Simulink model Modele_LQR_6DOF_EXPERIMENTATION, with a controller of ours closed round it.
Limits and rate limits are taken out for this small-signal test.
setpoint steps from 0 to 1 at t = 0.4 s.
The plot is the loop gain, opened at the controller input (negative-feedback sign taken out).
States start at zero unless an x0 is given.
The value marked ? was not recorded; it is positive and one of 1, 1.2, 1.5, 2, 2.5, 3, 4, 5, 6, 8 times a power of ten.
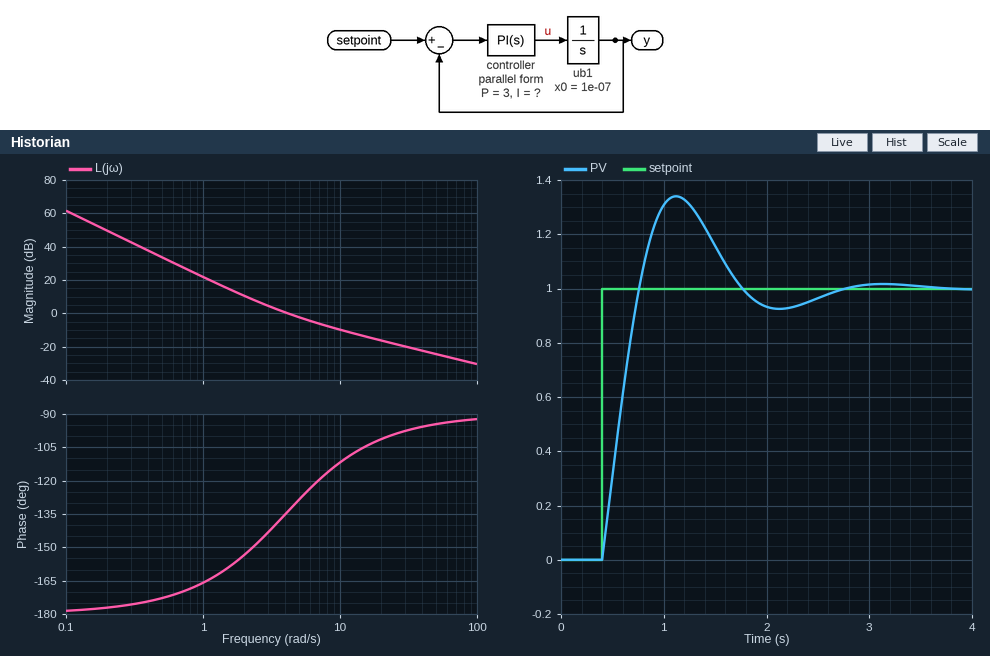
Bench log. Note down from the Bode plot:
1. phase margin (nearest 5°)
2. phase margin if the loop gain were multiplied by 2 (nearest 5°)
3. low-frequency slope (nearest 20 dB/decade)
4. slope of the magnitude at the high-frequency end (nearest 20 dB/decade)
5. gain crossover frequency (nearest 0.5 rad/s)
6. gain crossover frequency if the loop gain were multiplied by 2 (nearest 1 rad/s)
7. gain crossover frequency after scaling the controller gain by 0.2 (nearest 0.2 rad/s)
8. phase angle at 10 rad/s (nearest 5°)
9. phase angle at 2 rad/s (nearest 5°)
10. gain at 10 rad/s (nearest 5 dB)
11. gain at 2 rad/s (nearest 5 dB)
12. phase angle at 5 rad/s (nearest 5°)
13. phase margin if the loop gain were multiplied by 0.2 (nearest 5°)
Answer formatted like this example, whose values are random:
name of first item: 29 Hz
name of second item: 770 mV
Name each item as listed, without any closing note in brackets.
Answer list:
phase margin: 45°
phase margin if the loop gain were multiplied by 2: 60°
low-frequency slope: -40 dB/decade
slope of the magnitude at the high-frequency end: -20 dB/decade
gain crossover frequency: 4.0 rad/s
gain crossover frequency if the loop gain were multiplied by 2: 7 rad/s
gain crossover frequency after scaling the controller gain by 0.2: 1.6 rad/s
phase angle at 10 rad/s: -110°
phase angle at 2 rad/s: -155°
gain at 10 rad/s: -10 dB
gain at 2 rad/s: 10 dB
phase angle at 5 rad/s: -130°
phase margin if the loop gain were multiplied by 0.2: 20°
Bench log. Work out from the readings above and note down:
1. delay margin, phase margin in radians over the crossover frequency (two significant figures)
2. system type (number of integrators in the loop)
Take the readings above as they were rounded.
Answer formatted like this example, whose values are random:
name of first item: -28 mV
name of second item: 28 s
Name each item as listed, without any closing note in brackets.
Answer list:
delay margin, phase margin in radians over the crossover frequency: 0.20 s
system type: 2
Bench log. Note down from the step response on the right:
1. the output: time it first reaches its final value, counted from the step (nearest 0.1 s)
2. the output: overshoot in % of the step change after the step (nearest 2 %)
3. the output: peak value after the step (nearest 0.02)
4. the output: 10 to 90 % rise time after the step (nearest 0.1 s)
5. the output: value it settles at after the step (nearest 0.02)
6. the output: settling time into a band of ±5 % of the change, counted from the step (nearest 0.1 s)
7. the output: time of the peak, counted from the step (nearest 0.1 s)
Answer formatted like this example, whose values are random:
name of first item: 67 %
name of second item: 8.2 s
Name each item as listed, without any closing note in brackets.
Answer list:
the output: time it first reaches its final value, counted from the step: 0.4 s
the output: overshoot in % of the step change after the step: 34 %
the output: peak value after the step: 1.34
the output: 10 to 90 % rise time after the step: 0.3 s
the output: value it settles at after the step: 1.00
the output: settling time into a band of ±5 % of the change, counted from the step: 2.0 s
the output: time of the peak, counted from the step: 0.7 s
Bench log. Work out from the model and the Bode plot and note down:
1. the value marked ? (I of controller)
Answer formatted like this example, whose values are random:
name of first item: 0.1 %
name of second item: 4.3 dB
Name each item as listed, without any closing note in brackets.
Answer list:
the value marked ?: 12
